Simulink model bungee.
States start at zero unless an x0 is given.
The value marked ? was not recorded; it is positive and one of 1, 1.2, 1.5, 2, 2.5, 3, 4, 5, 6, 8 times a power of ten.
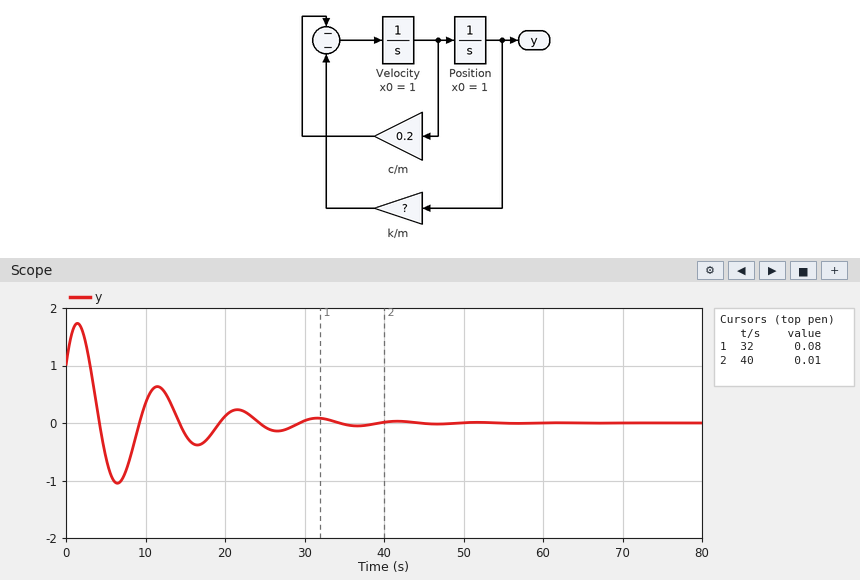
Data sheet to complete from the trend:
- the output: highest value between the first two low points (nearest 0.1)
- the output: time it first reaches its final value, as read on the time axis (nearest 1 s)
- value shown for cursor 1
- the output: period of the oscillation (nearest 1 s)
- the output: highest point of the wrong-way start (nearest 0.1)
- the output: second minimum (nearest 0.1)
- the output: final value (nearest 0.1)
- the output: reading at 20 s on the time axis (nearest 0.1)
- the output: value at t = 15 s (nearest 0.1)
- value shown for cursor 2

0.6
4 s
0.08
10 s
1.7
-0.4
0.0
0.1
-0.2
0.01
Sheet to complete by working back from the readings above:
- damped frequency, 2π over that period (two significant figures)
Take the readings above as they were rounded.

0.63 rad/s
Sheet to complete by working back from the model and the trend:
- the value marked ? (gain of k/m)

0.4
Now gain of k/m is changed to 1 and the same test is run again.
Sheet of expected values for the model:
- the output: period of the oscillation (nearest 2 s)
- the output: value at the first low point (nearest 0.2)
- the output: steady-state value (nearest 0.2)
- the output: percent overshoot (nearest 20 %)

6 s
-1.0
0.0
100 %
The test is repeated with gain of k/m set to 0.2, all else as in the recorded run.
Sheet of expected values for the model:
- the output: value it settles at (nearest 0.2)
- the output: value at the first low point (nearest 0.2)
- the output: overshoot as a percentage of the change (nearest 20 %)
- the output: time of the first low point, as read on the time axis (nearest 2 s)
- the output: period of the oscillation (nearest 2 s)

0.0
-1.0
100 %
10 s
14 s
